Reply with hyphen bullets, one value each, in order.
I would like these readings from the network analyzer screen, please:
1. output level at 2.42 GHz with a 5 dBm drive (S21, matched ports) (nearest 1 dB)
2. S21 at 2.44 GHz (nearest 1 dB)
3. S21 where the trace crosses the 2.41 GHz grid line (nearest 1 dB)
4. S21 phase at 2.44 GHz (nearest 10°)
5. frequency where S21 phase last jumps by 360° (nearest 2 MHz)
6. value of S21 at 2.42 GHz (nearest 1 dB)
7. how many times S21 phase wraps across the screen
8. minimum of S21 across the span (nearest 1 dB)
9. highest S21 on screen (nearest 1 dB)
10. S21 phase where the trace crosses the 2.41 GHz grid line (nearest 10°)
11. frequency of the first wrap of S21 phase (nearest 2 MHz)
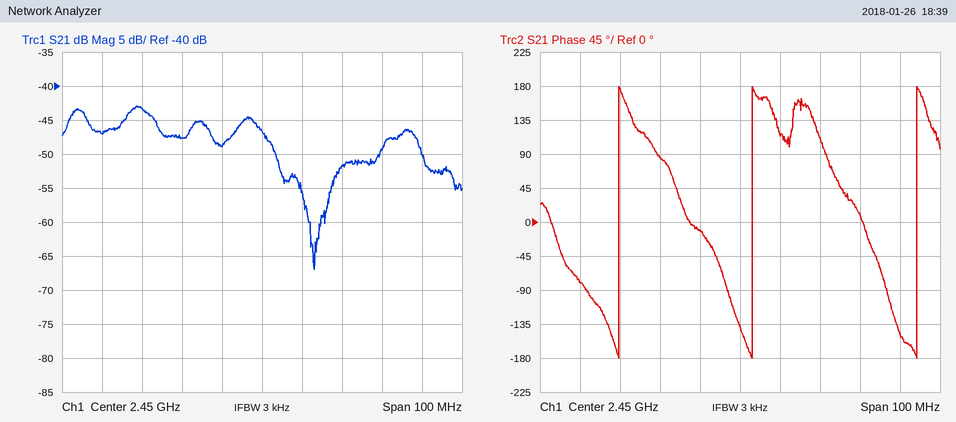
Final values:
- -38 dBm
- -49 dB
- -47 dB
- -10°
- 2.494 GHz
- -43 dB
- 3
- -67 dB
- -43 dB
- -80°
- 2.420 GHz
